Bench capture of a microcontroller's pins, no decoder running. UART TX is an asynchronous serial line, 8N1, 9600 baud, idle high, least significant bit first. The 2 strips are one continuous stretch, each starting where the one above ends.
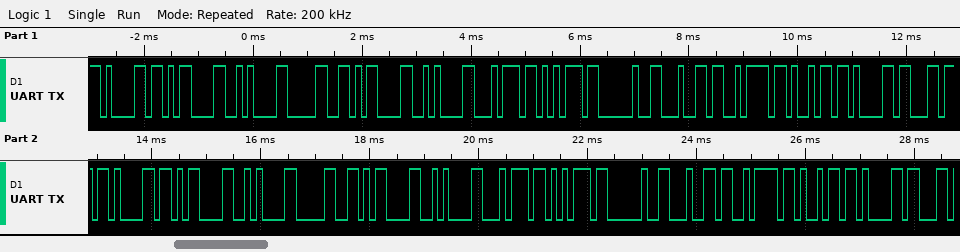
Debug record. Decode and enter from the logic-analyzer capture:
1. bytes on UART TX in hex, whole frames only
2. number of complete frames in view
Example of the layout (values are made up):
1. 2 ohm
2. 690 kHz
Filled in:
1. 0x61 0x0D 0x0A 0x30 0x0D 0x0A 0x74 0x75 0x20 0x64 0x7A 0x69 0x61 0x6C 0x61 0x0D 0x0A 0x30 0x0D 0x0A 0x74 0x75 0x20 0x64 0x7A 0x69 0x61
2. 27
